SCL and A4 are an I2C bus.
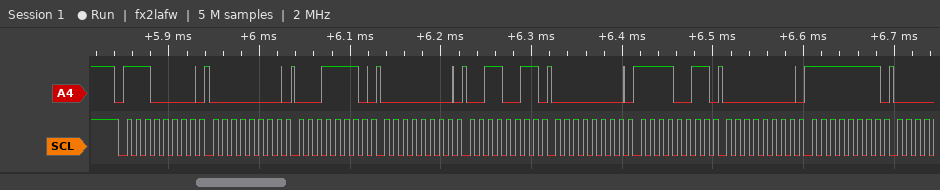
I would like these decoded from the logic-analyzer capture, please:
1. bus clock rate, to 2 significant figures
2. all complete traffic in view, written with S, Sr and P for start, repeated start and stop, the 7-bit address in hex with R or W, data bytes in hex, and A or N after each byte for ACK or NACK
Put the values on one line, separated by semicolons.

100 kHz; S 70W A 00 A 1E A 00 A 33 A 00 A F3 A 00 A FF A
